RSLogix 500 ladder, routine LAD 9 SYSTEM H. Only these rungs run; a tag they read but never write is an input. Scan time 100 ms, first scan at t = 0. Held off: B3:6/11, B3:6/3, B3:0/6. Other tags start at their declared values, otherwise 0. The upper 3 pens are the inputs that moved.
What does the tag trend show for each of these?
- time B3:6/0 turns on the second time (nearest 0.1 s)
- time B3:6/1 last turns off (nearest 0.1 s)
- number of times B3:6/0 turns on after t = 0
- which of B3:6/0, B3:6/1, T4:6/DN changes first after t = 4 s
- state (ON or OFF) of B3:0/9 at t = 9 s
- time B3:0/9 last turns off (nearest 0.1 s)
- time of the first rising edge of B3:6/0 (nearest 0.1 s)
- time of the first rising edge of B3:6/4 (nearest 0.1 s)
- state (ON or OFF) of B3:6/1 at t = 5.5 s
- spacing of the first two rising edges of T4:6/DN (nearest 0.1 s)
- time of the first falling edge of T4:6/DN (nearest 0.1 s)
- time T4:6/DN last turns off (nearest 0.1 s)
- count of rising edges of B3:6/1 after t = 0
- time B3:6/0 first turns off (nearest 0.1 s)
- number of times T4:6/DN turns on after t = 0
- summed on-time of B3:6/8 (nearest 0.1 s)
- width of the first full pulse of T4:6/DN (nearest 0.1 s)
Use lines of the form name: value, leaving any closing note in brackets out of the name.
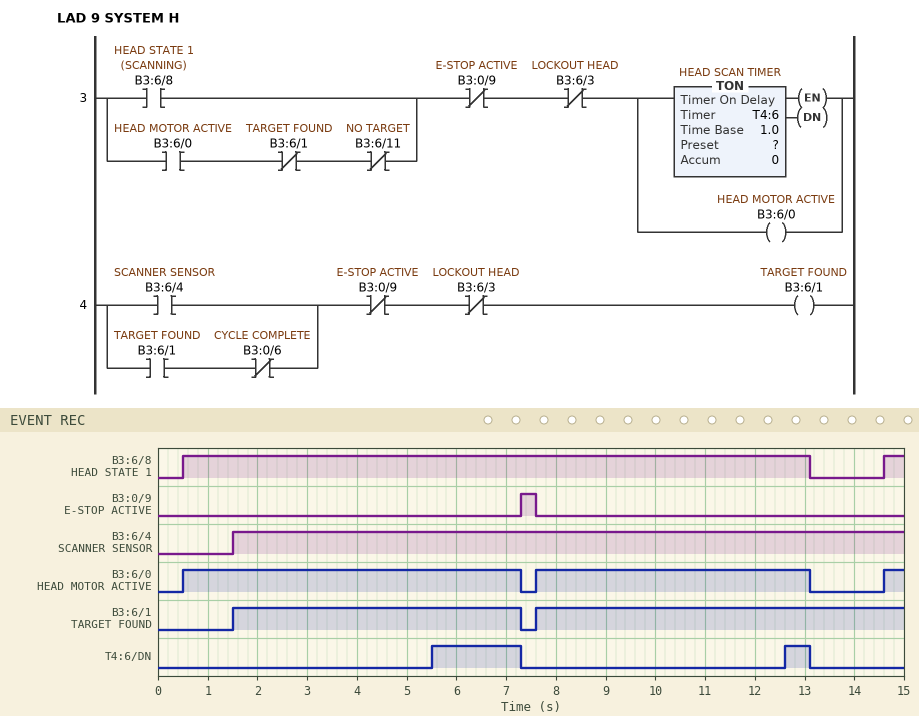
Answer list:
time B3:6/0 turns on the second time: 7.6 s
time B3:6/1 last turns off: 7.3 s
number of times B3:6/0 turns on after t = 0: 3
which of B3:6/0, B3:6/1, T4:6/DN changes first after t = 4 s: T4:6/DN
state (ON or OFF) of B3:0/9 at t = 9 s: OFF
time B3:0/9 last turns off: 7.6 s
time of the first rising edge of B3:6/0: 0.5 s
time of the first rising edge of B3:6/4: 1.5 s
state (ON or OFF) of B3:6/1 at t = 5.5 s: ON
spacing of the first two rising edges of T4:6/DN: 7.1 s
time of the first falling edge of T4:6/DN: 7.3 s
time T4:6/DN last turns off: 13.1 s
count of rising edges of B3:6/1 after t = 0: 2
time B3:6/0 first turns off: 7.3 s
number of times T4:6/DN turns on after t = 0: 2
summed on-time of B3:6/8: 13.0 s
width of the first full pulse of T4:6/DN: 1.8 s
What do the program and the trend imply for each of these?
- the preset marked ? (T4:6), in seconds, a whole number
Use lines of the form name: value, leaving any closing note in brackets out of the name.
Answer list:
the preset marked ? (T4:6), in seconds, a whole number: 5 s
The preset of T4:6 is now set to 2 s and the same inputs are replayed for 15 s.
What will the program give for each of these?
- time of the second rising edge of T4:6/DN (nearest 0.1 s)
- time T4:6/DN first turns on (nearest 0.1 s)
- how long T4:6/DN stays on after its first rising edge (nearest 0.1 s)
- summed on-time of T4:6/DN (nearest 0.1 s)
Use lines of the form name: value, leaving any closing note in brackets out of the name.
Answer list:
time of the second rising edge of T4:6/DN: 9.6 s
time T4:6/DN first turns on: 2.5 s
how long T4:6/DN stays on after its first rising edge: 4.8 s
summed on-time of T4:6/DN: 8.3 s
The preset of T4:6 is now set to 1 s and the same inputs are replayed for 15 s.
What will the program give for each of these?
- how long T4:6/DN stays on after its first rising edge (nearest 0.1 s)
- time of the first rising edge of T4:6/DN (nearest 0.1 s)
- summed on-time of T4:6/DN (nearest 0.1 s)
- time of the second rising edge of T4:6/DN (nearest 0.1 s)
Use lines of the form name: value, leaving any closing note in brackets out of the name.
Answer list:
how long T4:6/DN stays on after its first rising edge: 5.8 s
time of the first rising edge of T4:6/DN: 1.5 s
summed on-time of T4:6/DN: 10.3 s
time of the second rising edge of T4:6/DN: 8.6 s
